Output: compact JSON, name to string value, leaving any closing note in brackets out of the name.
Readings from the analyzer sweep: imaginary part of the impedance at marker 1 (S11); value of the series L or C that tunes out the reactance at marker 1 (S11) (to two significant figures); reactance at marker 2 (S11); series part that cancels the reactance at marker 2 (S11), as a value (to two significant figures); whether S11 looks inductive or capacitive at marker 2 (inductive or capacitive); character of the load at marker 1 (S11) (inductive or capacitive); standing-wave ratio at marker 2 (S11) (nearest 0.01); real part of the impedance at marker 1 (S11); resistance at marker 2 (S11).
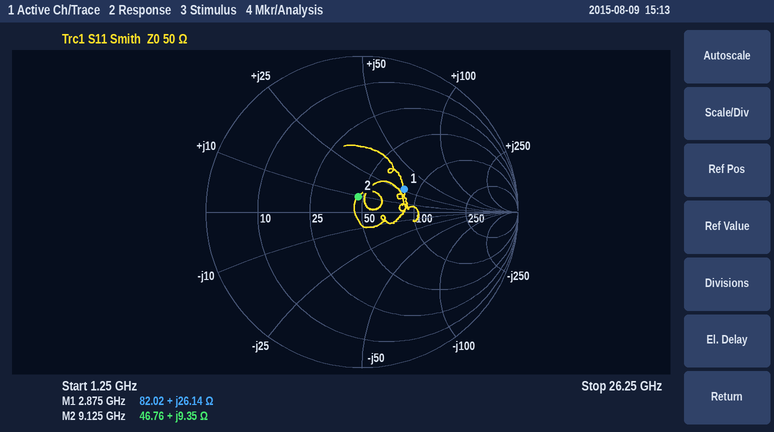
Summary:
{"imaginary part of the impedance at marker 1": "+26.14 Ω", "value of the series L or C that tunes out the reactance at marker 1 (S11)": "2.1 pF", "reactance at marker 2": "+9.35 Ω", "series part that cancels the reactance at marker 2 (S11), as a value": "1.9 pF", "whether S11 looks inductive or capacitive at marker 2": "inductive", "character of the load at marker 1 (S11)": "inductive", "standing-wave ratio at marker 2 (S11)": "1.23", "real part of the impedance at marker 1": "82.02 Ω", "resistance at marker 2": "46.76 Ω"}
